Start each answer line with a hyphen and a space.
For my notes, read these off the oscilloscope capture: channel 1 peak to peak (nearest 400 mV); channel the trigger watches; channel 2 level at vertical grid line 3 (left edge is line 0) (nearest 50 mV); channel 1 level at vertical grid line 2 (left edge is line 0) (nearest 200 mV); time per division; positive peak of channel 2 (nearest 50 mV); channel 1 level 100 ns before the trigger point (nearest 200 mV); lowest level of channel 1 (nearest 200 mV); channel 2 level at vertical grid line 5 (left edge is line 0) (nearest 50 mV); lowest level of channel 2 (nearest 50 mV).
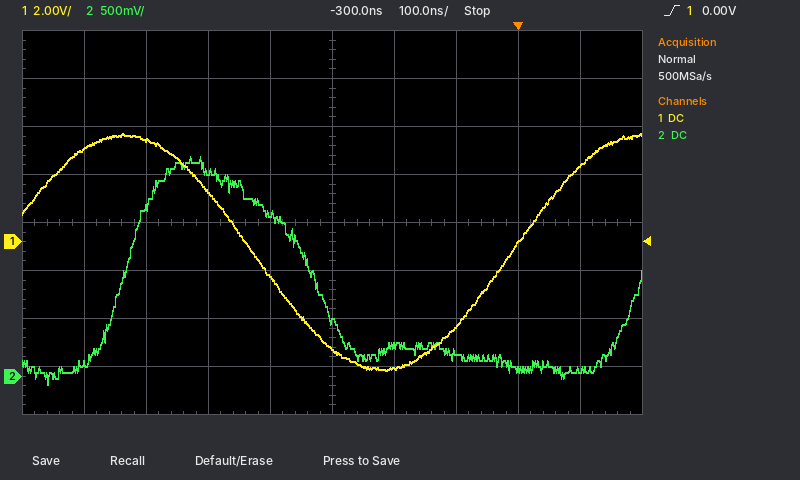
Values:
- 10.0 V
- channel 1
- 2.15 V
- 4.2 V
- 100 ns
- 2.30 V
- -3.6 V
- -5.4 V
- 600 mV
- -100 mV
